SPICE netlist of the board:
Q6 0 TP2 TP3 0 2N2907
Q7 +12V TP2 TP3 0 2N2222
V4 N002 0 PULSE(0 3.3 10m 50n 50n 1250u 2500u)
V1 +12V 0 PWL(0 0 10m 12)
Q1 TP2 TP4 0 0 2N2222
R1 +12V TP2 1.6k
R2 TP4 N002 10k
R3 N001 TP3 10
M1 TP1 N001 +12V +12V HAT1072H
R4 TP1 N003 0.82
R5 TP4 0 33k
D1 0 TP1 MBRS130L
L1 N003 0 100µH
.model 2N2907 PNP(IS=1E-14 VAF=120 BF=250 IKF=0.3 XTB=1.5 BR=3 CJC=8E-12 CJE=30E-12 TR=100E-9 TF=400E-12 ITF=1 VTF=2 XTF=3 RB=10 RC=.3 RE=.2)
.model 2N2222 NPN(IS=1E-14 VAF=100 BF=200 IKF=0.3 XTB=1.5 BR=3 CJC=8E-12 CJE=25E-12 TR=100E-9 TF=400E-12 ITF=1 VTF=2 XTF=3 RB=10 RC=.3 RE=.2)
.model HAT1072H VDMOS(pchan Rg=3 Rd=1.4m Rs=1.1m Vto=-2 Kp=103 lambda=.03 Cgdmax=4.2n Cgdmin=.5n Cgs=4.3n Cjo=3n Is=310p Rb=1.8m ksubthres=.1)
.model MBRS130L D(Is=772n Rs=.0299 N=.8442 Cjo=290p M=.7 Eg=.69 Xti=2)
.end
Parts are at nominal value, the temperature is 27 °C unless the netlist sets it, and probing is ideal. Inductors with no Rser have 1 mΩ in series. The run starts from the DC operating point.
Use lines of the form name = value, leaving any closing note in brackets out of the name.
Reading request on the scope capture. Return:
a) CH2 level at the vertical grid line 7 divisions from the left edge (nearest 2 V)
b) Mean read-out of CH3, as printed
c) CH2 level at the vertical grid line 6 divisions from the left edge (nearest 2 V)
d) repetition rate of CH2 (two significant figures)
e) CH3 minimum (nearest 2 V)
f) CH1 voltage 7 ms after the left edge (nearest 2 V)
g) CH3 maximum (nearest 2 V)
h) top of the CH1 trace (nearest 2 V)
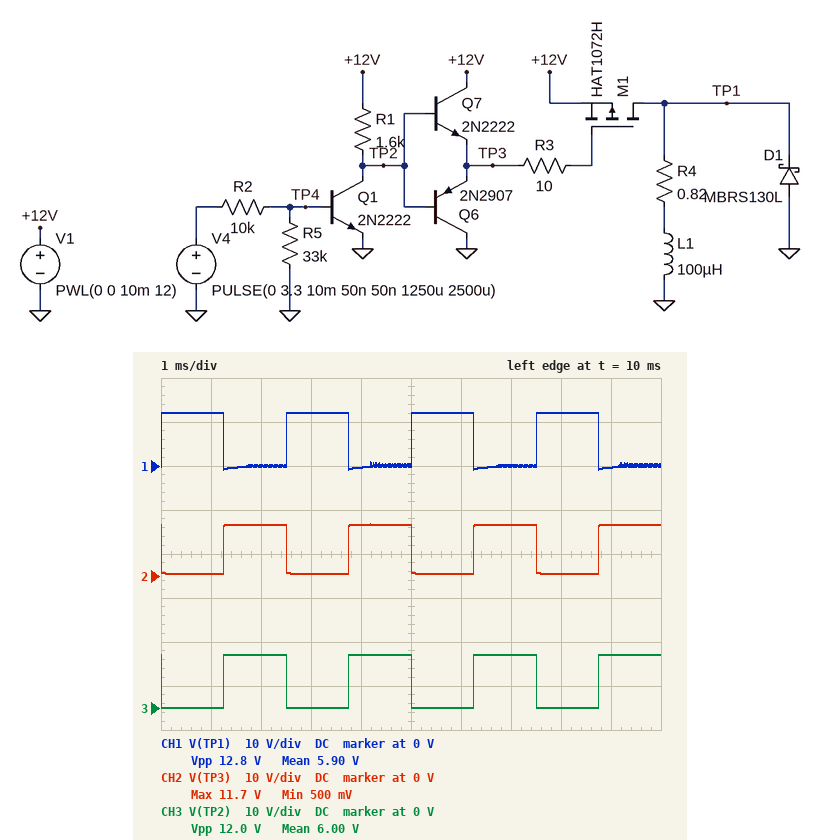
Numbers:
CH2 level at the vertical grid line 7 divisions from the left edge = 12 V
Mean read-out of CH3, as printed = 6.00 V
CH2 level at the vertical grid line 6 divisions from the left edge = 0 V
repetition rate of CH2 = 400 Hz
CH3 minimum = 0 V
CH1 voltage 7 ms after the left edge = 0 V
CH3 maximum = 12 V
top of the CH1 trace = 12 V
